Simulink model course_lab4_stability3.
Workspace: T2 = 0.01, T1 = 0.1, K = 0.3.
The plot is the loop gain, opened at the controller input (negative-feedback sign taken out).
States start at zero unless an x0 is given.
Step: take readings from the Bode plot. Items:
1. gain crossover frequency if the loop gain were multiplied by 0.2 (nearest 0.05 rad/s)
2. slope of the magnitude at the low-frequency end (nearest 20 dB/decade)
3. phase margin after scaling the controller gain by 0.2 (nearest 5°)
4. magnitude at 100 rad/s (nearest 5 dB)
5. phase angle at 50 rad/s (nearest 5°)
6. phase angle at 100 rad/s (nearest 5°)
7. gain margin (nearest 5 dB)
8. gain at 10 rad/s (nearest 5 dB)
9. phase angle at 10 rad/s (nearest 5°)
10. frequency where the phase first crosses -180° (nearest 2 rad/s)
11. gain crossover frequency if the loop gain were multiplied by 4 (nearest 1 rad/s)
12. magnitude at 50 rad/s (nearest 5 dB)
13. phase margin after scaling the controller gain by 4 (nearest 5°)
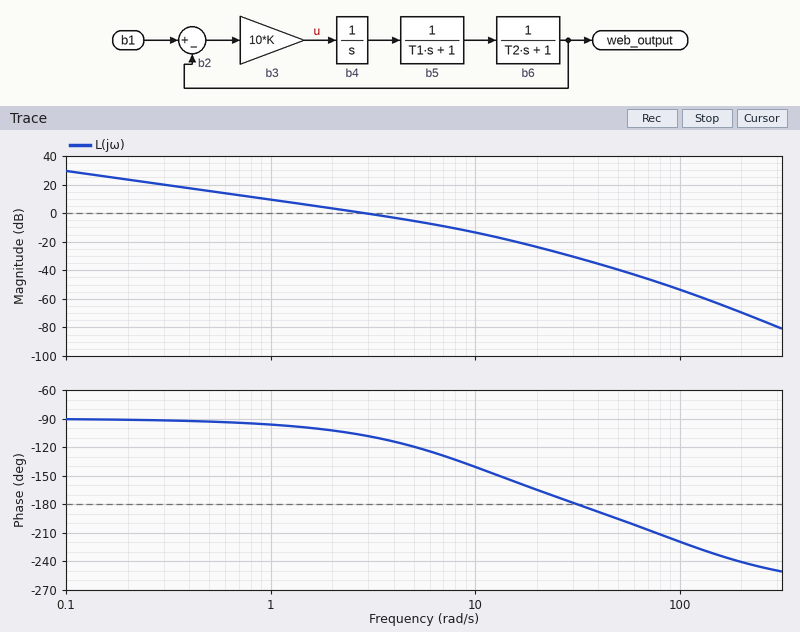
0.60 rad/s
-20 dB/decade
85°
-55 dB
-195°
-220°
30 dB
-15 dB
-140°
32 rad/s
9 rad/s
-40 dB
45°
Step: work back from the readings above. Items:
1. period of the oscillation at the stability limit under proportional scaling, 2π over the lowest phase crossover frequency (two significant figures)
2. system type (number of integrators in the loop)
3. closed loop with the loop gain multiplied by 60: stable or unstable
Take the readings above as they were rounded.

0.20 s
1
unstable
